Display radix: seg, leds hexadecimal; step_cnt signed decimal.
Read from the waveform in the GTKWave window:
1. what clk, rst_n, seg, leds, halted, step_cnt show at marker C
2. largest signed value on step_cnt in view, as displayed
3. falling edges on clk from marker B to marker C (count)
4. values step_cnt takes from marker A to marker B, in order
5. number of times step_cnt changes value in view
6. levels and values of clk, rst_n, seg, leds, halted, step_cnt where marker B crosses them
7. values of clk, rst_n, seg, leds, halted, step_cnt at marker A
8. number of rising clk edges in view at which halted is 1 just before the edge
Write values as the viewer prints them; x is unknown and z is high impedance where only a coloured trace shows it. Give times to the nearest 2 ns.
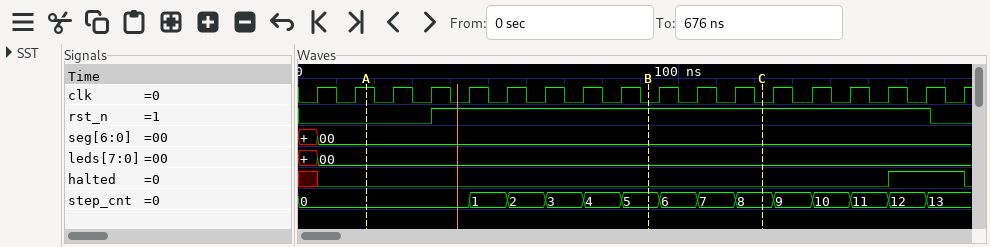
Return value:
clk=0, rst_n=1, seg=00, leds=00, halted=0, step_cnt=8
13
3
0, 1, 2, 3, 4, 5
13
clk=0, rst_n=1, seg=00, leds=00, halted=0, step_cnt=5
clk=1, rst_n=0, seg=00, leds=00, halted=0, step_cnt=0
2
